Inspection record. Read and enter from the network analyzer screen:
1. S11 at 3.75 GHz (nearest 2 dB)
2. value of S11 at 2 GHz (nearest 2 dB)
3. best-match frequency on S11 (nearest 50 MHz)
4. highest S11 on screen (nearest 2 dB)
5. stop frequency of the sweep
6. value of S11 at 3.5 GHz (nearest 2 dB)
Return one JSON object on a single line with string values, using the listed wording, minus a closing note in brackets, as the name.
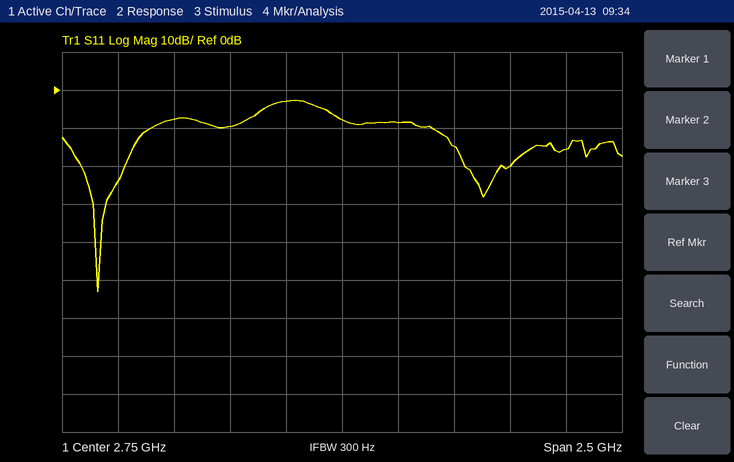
{"S11 at 3.75 GHz": "-16 dB", "value of S11 at 2 GHz": "-8 dB", "best-match frequency on S11": "1.65 GHz", "highest S11 on screen": "-2 dB", "stop frequency of the sweep": "4 GHz", "value of S11 at 3.5 GHz": "-20 dB"}
